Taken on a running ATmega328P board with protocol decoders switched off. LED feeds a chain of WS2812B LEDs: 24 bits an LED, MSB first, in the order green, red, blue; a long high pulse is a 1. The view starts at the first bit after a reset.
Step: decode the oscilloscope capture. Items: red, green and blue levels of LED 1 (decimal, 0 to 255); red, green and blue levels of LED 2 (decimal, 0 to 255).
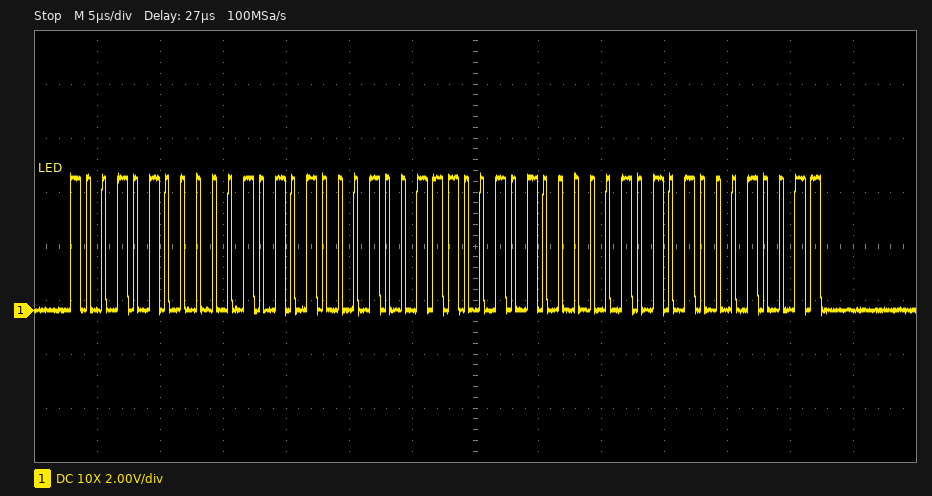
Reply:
21, 148, 19
21, 148, 19
